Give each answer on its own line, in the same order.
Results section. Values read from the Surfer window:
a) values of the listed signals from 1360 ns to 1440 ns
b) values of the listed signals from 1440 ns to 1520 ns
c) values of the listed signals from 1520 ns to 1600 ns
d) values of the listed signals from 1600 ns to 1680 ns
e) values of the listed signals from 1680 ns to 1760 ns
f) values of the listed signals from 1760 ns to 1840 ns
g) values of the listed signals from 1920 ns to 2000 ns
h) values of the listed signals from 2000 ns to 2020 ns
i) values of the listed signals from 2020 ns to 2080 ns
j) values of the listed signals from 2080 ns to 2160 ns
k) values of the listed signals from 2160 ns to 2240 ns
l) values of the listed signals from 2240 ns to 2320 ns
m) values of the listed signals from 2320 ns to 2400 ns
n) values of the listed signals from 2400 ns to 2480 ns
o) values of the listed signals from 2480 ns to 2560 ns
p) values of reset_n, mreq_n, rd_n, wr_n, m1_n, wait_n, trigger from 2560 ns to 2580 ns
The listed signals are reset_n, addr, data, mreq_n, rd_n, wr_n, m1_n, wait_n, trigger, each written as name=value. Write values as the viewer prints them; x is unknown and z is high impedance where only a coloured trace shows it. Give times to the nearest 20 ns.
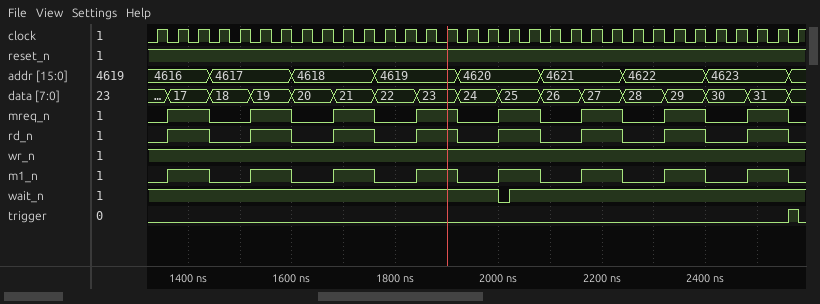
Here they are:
reset_n=1, addr=4616, data=17, mreq_n=1, rd_n=1, wr_n=1, m1_n=1, wait_n=1, trigger=0
reset_n=1, addr=4617, data=18, mreq_n=0, rd_n=0, wr_n=1, m1_n=0, wait_n=1, trigger=0
reset_n=1, addr=4617, data=19, mreq_n=1, rd_n=1, wr_n=1, m1_n=1, wait_n=1, trigger=0
reset_n=1, addr=4618, data=20, mreq_n=0, rd_n=0, wr_n=1, m1_n=0, wait_n=1, trigger=0
reset_n=1, addr=4618, data=21, mreq_n=1, rd_n=1, wr_n=1, m1_n=1, wait_n=1, trigger=0
reset_n=1, addr=4619, data=22, mreq_n=0, rd_n=0, wr_n=1, m1_n=0, wait_n=1, trigger=0
reset_n=1, addr=4620, data=24, mreq_n=0, rd_n=0, wr_n=1, m1_n=0, wait_n=1, trigger=0
reset_n=1, addr=4620, data=25, mreq_n=1, rd_n=1, wr_n=1, m1_n=1, wait_n=0, trigger=0
reset_n=1, addr=4620, data=25, mreq_n=1, rd_n=1, wr_n=1, m1_n=1, wait_n=1, trigger=0
reset_n=1, addr=4621, data=26, mreq_n=0, rd_n=0, wr_n=1, m1_n=0, wait_n=1, trigger=0
reset_n=1, addr=4621, data=27, mreq_n=1, rd_n=1, wr_n=1, m1_n=1, wait_n=1, trigger=0
reset_n=1, addr=4622, data=28, mreq_n=0, rd_n=0, wr_n=1, m1_n=0, wait_n=1, trigger=0
reset_n=1, addr=4622, data=29, mreq_n=1, rd_n=1, wr_n=1, m1_n=1, wait_n=1, trigger=0
reset_n=1, addr=4623, data=30, mreq_n=0, rd_n=0, wr_n=1, m1_n=0, wait_n=1, trigger=0
reset_n=1, addr=4623, data=31, mreq_n=1, rd_n=1, wr_n=1, m1_n=1, wait_n=1, trigger=0
reset_n=1, mreq_n=0, rd_n=0, wr_n=1, m1_n=0, wait_n=1, trigger=1
